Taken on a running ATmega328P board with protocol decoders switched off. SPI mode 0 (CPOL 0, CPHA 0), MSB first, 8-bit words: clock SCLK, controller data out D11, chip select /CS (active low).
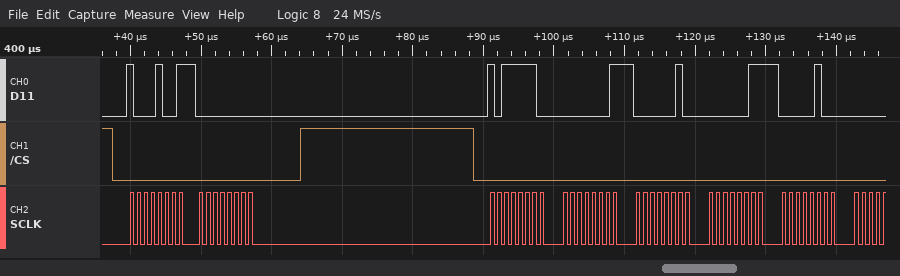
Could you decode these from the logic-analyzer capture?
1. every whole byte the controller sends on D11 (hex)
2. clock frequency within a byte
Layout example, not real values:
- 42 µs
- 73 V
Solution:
- 89 00 BE 01 02 03 04
- 1 MHz
